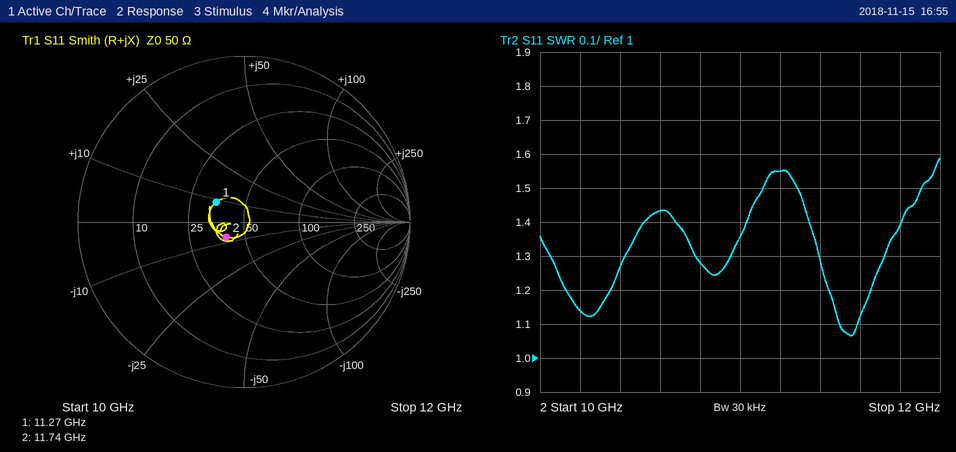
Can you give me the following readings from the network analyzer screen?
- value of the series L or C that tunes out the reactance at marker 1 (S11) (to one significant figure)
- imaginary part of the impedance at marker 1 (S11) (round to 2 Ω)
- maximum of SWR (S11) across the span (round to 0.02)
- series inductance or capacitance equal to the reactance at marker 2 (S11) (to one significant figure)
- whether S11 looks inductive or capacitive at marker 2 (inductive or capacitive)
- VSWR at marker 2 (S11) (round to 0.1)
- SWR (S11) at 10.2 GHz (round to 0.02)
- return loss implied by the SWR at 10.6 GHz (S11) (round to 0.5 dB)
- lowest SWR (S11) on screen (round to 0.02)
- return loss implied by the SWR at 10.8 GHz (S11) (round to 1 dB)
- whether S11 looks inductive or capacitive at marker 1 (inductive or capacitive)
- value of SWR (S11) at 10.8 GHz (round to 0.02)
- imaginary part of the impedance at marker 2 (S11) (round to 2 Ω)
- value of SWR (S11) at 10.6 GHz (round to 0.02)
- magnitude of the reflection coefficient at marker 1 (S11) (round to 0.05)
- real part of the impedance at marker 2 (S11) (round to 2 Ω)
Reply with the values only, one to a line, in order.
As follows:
2 pF
+8 Ω
1.58
2 pF
capacitive
1.3
1.14
15.0 dB
1.06
18 dB
inductive
1.28
-8 Ω
1.44
0.20
40 Ω
